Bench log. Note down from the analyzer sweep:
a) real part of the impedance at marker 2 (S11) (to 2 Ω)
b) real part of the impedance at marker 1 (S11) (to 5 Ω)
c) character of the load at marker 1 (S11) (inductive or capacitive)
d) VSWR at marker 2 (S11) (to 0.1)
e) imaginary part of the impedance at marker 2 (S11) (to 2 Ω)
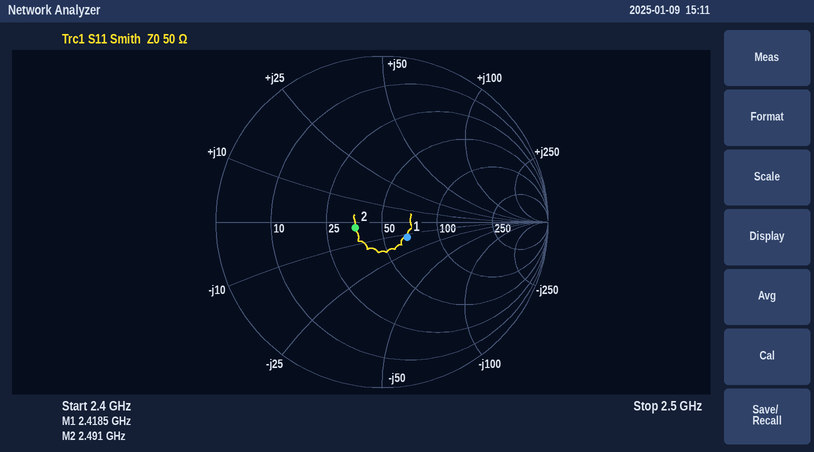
36 Ω
65 Ω
capacitive
1.4
-2 Ω
